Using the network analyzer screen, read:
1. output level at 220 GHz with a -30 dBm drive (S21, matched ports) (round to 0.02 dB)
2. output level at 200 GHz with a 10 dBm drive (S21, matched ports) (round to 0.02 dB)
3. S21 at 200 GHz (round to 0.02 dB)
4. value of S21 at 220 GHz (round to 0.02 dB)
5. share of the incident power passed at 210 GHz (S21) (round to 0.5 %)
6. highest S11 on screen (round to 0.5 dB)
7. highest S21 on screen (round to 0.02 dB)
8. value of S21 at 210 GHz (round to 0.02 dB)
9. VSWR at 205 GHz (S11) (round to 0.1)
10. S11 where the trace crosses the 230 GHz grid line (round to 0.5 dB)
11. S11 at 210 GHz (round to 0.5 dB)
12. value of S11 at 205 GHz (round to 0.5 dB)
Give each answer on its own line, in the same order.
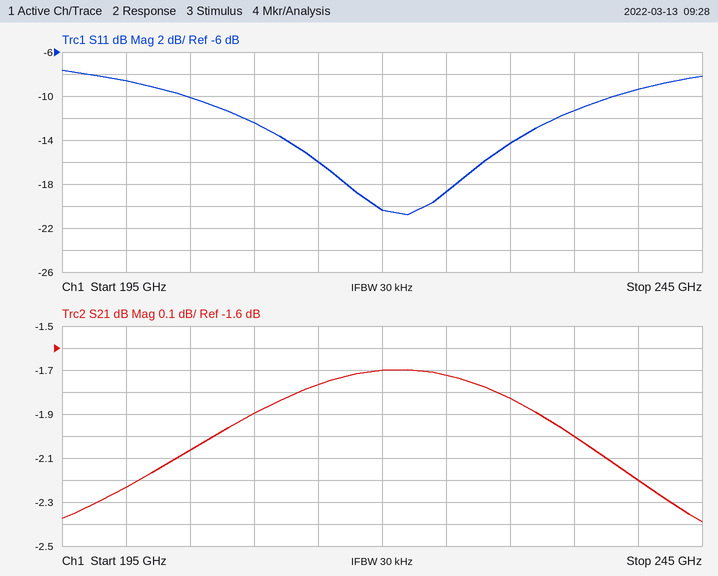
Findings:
-31.70 dBm
7.76 dBm
-2.24 dB
-1.70 dB
64.5 %
-7.5 dB
-1.70 dB
-1.90 dB
1.9
-14.5 dB
-12.5 dB
-10.0 dB
